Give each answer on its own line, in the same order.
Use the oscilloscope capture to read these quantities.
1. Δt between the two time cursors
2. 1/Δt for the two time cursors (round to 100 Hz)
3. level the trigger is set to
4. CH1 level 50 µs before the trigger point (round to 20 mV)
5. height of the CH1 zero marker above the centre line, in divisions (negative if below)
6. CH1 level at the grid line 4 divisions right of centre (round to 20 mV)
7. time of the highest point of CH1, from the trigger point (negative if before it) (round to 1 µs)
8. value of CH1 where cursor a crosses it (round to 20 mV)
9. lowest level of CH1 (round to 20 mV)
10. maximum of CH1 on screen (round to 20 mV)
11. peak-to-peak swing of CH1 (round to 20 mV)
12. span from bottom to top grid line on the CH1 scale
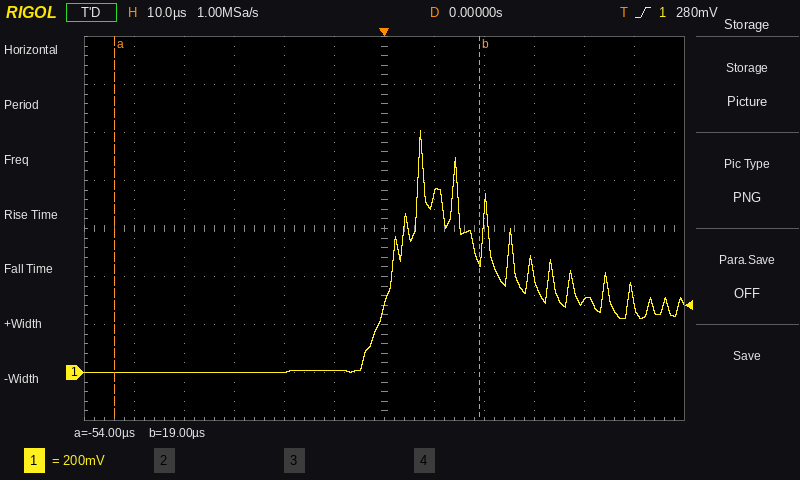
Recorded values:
73 µs
13.7 kHz
280 mV
0 mV
-3.0 div
300 mV
+7 µs
0 mV
0 mV
1.00 V
1.00 V
1.6 V
